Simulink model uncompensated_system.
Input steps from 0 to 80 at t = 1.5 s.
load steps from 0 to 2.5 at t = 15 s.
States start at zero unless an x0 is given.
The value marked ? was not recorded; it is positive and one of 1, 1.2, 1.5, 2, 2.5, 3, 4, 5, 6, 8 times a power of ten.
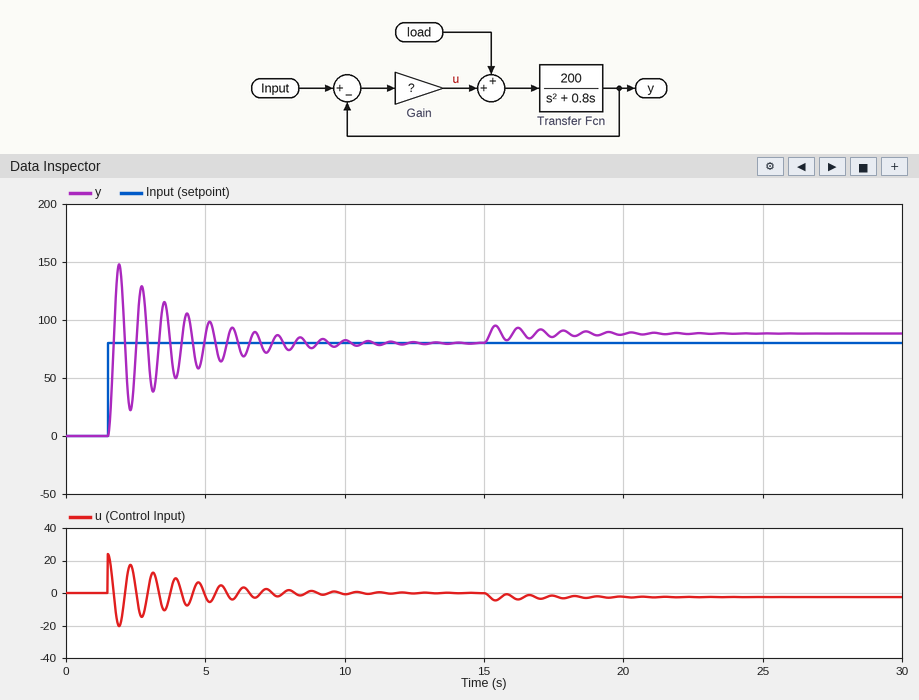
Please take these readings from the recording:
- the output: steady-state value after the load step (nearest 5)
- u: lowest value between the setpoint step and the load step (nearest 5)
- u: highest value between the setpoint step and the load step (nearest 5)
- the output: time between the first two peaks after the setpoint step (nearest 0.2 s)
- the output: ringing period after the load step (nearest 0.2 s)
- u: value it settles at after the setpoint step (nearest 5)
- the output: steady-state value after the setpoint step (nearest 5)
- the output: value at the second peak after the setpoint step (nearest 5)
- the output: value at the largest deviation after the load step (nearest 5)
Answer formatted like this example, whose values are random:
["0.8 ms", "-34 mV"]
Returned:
["90", "-20", "25", "0.8 s", "0.8 s", "0", "80", "130", "95"]
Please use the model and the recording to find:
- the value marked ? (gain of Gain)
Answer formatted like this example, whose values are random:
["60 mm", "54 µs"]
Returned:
["0.3"]
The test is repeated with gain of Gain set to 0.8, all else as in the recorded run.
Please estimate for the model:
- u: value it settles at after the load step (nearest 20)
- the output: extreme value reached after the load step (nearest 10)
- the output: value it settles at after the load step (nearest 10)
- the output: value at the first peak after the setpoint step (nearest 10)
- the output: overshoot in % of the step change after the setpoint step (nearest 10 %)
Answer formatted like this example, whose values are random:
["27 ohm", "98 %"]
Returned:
["0", "90", "80", "150", "90 %"]
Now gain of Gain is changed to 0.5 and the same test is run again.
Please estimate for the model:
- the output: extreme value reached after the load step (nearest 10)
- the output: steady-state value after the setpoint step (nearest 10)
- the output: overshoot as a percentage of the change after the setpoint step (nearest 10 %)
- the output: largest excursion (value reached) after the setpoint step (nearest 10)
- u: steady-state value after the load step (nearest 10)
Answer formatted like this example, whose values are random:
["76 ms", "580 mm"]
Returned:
["90", "80", "90 %", "150", "0"]
